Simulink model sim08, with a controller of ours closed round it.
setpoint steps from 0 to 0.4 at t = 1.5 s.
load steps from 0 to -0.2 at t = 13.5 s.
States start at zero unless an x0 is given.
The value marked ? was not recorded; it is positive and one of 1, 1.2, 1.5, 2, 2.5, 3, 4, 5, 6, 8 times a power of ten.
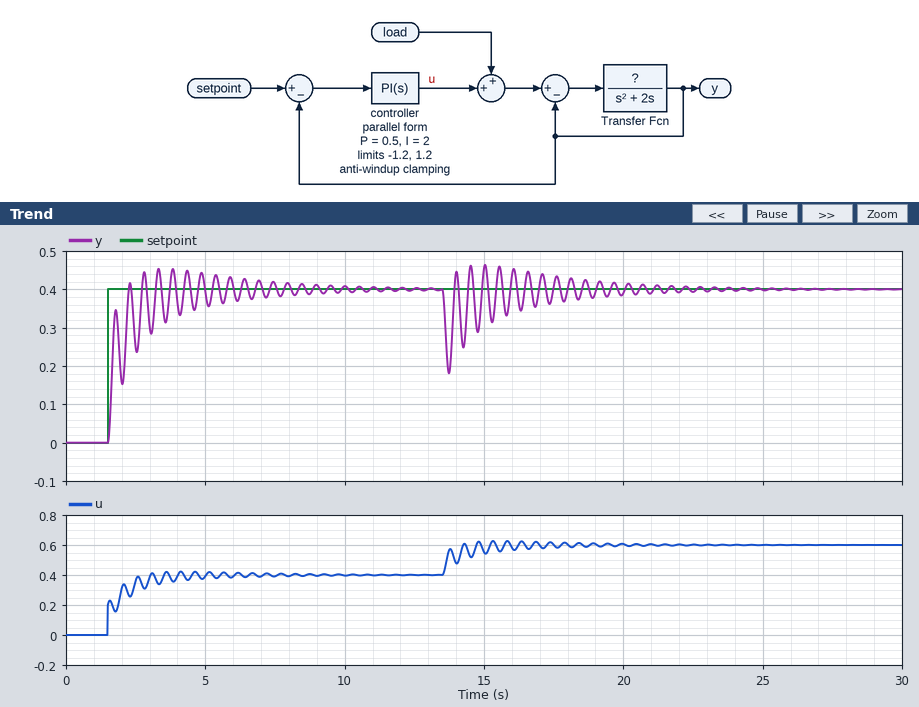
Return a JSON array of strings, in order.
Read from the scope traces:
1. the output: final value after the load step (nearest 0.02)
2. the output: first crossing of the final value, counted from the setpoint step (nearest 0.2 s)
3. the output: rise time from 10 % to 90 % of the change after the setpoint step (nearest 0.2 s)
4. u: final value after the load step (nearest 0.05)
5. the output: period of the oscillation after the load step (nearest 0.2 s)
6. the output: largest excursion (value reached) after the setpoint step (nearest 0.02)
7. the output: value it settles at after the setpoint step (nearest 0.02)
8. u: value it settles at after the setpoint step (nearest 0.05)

["0.40", "0.8 s", "0.6 s", "0.60", "0.6 s", "0.46", "0.40", "0.40"]
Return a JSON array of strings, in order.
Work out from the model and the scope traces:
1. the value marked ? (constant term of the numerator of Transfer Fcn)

["100"]
